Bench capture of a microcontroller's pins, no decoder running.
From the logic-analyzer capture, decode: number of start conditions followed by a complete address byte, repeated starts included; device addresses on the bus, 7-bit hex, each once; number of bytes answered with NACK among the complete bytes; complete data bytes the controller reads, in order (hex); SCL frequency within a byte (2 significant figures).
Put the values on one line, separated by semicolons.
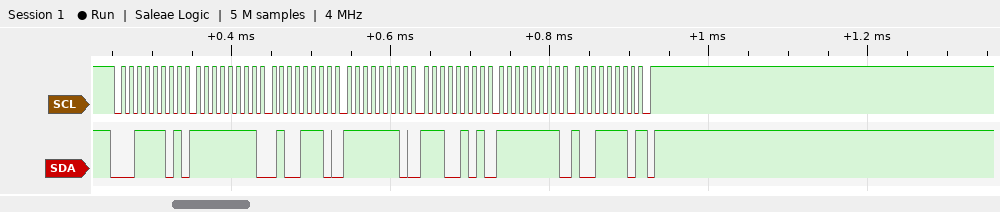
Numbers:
1; 0x1E; 1; FF 4E FE E5 FF 9E; 100 kHz
